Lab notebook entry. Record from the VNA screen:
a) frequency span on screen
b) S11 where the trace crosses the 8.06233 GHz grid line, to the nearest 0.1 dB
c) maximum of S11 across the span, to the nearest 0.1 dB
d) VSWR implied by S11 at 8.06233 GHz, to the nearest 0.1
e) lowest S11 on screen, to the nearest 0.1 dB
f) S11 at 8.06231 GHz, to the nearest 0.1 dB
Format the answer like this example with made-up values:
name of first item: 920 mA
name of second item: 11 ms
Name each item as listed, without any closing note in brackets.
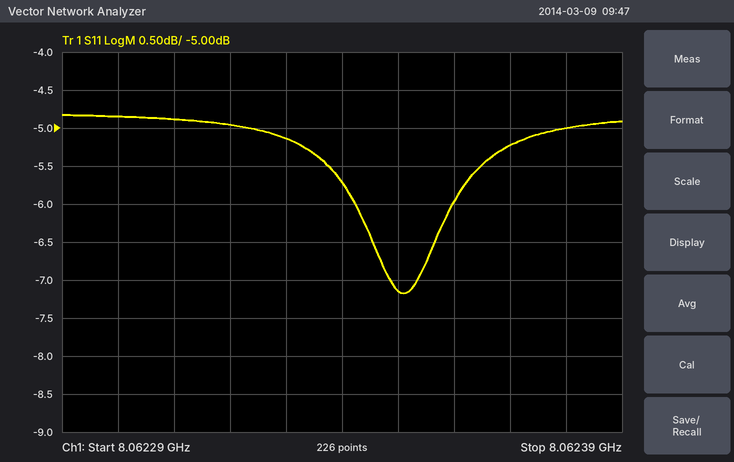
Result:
frequency span on screen: 100 kHz
S11 where the trace crosses the 8.06233 GHz grid line, to the nearest 0.1 dB: -5.1 dB
maximum of S11 across the span, to the nearest 0.1 dB: -4.8 dB
VSWR implied by S11 at 8.06233 GHz, to the nearest 0.1: 3.5
lowest S11 on screen, to the nearest 0.1 dB: -7.2 dB
S11 at 8.06231 GHz, to the nearest 0.1 dB: -4.9 dB
